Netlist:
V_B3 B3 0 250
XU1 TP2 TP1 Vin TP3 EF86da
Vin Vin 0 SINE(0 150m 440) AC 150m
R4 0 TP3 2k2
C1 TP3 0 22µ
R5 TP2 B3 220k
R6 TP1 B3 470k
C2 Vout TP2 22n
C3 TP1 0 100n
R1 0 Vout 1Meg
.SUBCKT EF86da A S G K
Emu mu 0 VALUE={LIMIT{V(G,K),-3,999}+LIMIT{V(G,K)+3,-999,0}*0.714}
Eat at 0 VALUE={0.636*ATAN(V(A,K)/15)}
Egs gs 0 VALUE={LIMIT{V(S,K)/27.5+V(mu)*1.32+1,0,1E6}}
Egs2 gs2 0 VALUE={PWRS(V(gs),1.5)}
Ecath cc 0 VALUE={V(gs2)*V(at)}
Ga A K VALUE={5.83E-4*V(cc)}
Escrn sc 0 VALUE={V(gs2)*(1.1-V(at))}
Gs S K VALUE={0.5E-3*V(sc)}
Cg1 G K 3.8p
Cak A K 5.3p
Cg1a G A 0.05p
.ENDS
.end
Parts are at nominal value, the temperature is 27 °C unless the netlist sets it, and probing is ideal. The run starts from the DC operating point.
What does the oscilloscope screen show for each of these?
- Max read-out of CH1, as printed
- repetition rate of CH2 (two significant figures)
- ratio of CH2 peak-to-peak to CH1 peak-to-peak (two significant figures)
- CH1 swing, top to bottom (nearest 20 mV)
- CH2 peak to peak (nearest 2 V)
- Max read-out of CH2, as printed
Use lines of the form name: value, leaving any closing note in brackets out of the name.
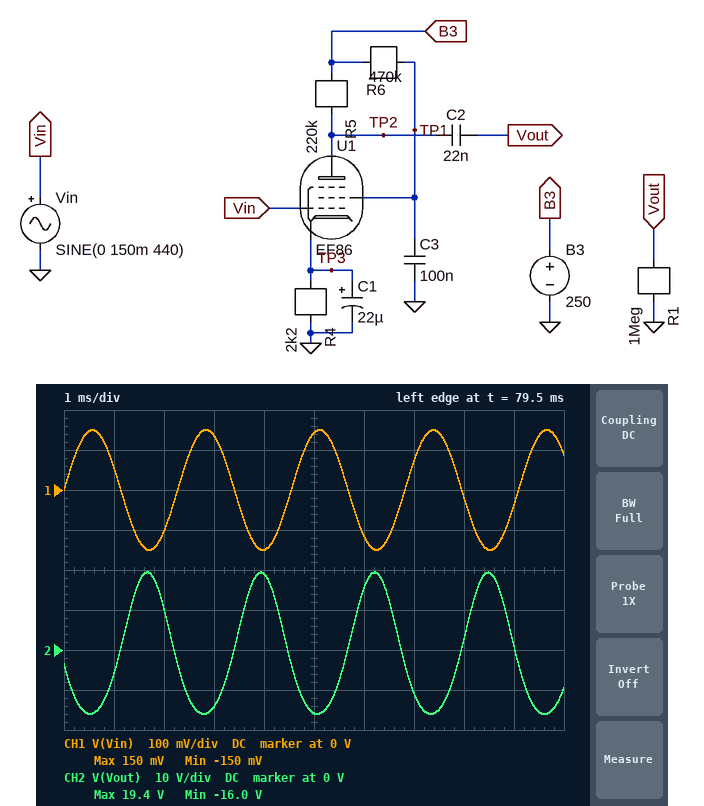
Max read-out of CH1, as printed: 150 mV
repetition rate of CH2: 440 Hz
ratio of CH2 peak-to-peak to CH1 peak-to-peak: 120
CH1 swing, top to bottom: 300 mV
CH2 peak to peak: 36 V
Max read-out of CH2, as printed: 19.4 V
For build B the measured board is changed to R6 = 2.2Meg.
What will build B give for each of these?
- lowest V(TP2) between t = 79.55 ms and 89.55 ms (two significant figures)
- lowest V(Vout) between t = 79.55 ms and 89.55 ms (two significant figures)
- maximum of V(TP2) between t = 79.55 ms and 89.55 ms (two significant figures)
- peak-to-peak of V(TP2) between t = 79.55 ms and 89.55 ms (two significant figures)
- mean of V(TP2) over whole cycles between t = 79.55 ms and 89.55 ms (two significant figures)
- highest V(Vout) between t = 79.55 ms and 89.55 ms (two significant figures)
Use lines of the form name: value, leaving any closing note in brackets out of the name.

lowest V(TP2) between t = 79.55 ms and 89.55 ms: 100 V
lowest V(Vout) between t = 79.55 ms and 89.55 ms: -27 V
maximum of V(TP2) between t = 79.55 ms and 89.55 ms: 160 V
peak-to-peak of V(TP2) between t = 79.55 ms and 89.55 ms: 54 V
mean of V(TP2) over whole cycles between t = 79.55 ms and 89.55 ms: 130 V
highest V(Vout) between t = 79.55 ms and 89.55 ms: 27 V
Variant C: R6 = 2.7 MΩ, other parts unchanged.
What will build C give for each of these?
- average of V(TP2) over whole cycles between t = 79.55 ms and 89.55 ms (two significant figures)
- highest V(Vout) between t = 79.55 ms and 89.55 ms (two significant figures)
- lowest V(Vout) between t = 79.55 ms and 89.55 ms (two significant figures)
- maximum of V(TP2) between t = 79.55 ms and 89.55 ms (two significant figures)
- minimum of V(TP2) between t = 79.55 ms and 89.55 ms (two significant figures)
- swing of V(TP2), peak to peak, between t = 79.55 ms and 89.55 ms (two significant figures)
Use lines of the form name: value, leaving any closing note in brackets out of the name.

average of V(TP2) over whole cycles between t = 79.55 ms and 89.55 ms: 140 V
highest V(Vout) between t = 79.55 ms and 89.55 ms: 26 V
lowest V(Vout) between t = 79.55 ms and 89.55 ms: -27 V
maximum of V(TP2) between t = 79.55 ms and 89.55 ms: 170 V
minimum of V(TP2) between t = 79.55 ms and 89.55 ms: 120 V
swing of V(TP2), peak to peak, between t = 79.55 ms and 89.55 ms: 53 V
